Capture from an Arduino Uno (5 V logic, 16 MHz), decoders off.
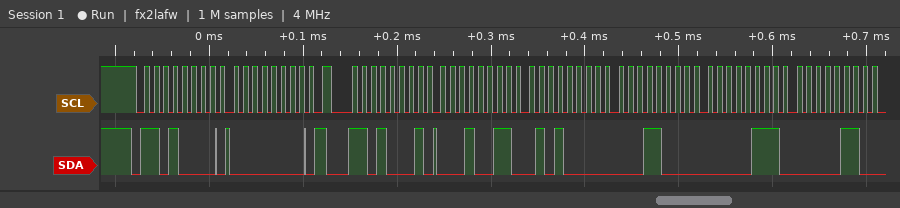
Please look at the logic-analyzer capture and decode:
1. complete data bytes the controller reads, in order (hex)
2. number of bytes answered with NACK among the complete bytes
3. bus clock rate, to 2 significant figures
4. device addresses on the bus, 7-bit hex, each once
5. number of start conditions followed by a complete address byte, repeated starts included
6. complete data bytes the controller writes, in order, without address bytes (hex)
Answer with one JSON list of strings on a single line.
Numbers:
["13 50 18 07 06", "0", "100 kHz", "0x68", "2", "00"]
